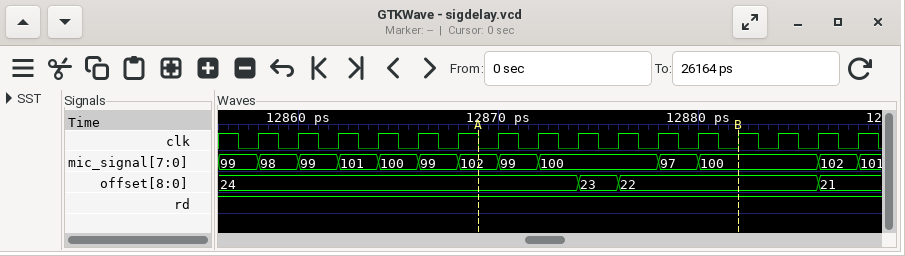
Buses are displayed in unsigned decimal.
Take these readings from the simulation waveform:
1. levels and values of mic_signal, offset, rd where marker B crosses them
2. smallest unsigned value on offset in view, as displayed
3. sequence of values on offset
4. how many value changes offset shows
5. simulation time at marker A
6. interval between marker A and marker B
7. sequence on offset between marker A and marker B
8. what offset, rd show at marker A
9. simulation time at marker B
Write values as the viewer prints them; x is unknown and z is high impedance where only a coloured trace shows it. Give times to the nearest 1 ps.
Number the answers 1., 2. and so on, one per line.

1. mic_signal=100, offset=22, rd=1
2. 21
3. 24, 23, 22, 21
4. 3
5. 12869 ps
6. 13 ps
7. 24, 23, 22
8. offset=24, rd=1
9. 12882 ps
